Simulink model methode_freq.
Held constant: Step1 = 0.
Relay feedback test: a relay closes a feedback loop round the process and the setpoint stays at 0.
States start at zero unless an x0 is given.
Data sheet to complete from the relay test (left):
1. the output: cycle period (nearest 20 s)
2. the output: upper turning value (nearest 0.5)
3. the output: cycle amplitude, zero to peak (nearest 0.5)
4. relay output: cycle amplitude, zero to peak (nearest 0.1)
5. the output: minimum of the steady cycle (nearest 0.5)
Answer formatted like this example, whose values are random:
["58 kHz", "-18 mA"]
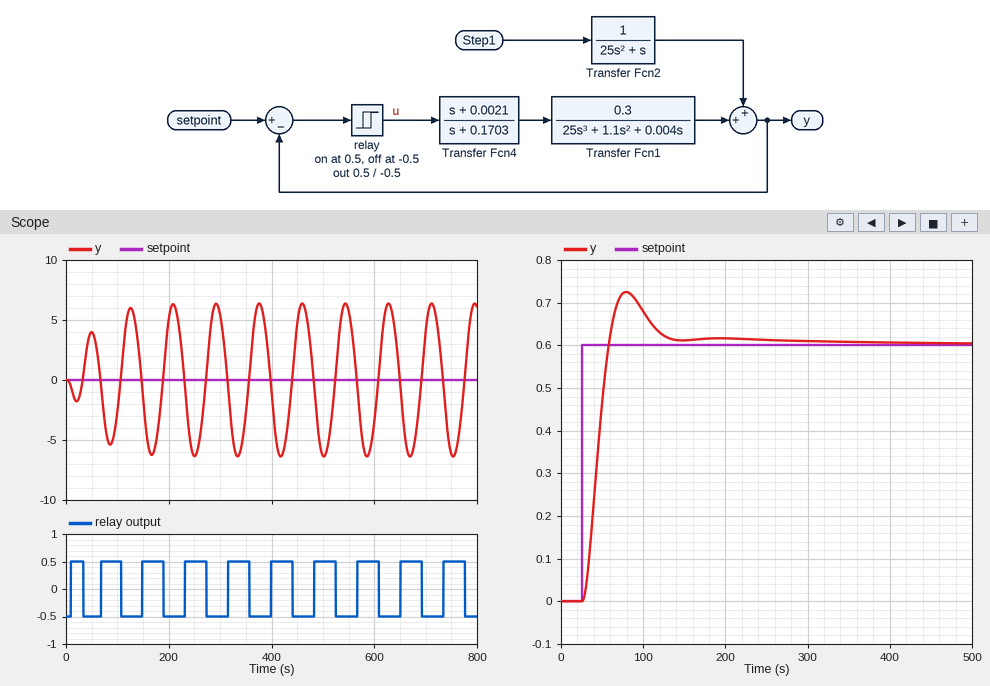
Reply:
["80 s", "6.5", "6.5", "0.5", "-6.5"]
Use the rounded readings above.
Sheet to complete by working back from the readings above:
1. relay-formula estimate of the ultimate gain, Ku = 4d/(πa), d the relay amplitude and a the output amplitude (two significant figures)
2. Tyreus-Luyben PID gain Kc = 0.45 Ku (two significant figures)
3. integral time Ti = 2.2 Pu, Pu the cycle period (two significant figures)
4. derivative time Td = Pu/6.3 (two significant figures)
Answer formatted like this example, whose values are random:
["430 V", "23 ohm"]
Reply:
["0.098", "0.044", "180 s", "13 s"]
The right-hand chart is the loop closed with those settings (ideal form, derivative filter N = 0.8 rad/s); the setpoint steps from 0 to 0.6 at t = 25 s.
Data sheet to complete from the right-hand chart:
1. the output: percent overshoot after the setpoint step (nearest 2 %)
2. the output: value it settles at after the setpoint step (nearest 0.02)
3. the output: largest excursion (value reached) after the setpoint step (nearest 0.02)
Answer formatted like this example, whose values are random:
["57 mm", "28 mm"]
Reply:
["20 %", "0.60", "0.72"]
